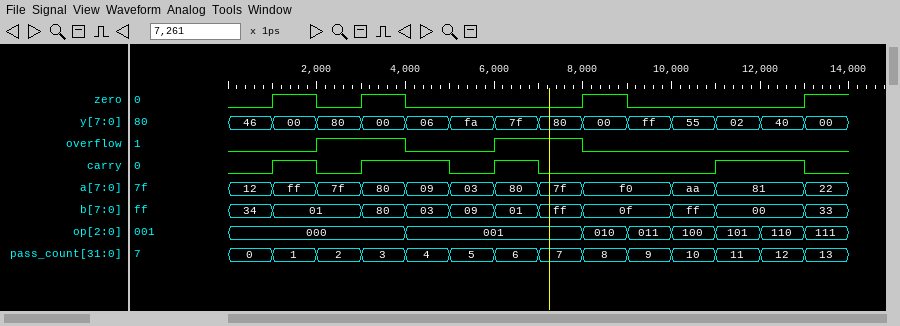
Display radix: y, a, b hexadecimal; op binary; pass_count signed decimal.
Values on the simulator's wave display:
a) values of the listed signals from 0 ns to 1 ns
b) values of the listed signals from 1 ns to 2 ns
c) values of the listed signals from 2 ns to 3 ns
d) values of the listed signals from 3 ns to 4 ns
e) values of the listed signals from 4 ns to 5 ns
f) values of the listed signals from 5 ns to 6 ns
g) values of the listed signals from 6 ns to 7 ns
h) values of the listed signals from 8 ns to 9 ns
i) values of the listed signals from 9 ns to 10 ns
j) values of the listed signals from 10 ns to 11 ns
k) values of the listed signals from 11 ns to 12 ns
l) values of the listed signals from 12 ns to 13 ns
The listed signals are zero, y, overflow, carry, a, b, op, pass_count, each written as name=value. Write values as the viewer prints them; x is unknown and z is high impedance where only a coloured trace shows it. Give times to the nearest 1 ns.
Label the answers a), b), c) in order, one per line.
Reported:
a) zero=0, y=46, overflow=0, carry=0, a=12, b=34, op=000, pass_count=0
b) zero=1, y=00, overflow=0, carry=1, a=ff, b=01, op=000, pass_count=1
c) zero=0, y=80, overflow=1, carry=0, a=7f, b=01, op=000, pass_count=2
d) zero=1, y=00, overflow=1, carry=1, a=80, b=80, op=000, pass_count=3
e) zero=0, y=06, overflow=0, carry=1, a=09, b=03, op=001, pass_count=4
f) zero=0, y=fa, overflow=0, carry=0, a=03, b=09, op=001, pass_count=5
g) zero=0, y=7f, overflow=1, carry=1, a=80, b=01, op=001, pass_count=6
h) zero=1, y=00, overflow=0, carry=0, a=f0, b=0f, op=010, pass_count=8
i) zero=0, y=ff, overflow=0, carry=0, a=f0, b=0f, op=011, pass_count=9
j) zero=0, y=55, overflow=0, carry=0, a=aa, b=ff, op=100, pass_count=10
k) zero=0, y=02, overflow=0, carry=1, a=81, b=00, op=101, pass_count=11
l) zero=0, y=40, overflow=0, carry=1, a=81, b=00, op=110, pass_count=12
